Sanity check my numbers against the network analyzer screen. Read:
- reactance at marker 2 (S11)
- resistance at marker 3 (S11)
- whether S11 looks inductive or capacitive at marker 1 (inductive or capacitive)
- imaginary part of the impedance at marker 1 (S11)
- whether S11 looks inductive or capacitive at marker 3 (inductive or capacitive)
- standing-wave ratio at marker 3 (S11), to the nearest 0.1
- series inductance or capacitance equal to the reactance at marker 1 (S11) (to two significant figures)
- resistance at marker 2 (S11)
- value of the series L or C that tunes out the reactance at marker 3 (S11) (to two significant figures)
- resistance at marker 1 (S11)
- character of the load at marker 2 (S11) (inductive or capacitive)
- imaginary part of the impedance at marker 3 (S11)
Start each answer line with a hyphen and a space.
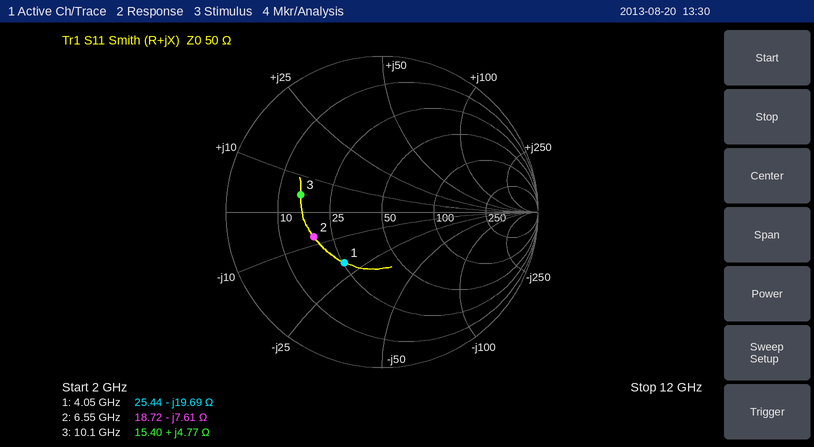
- -7.61 Ω
- 15.40 Ω
- capacitive
- -19.69 Ω
- inductive
- 3.3
- 2.0 pF
- 18.72 Ω
- 3.3 pF
- 25.44 Ω
- capacitive
- +4.77 Ω
